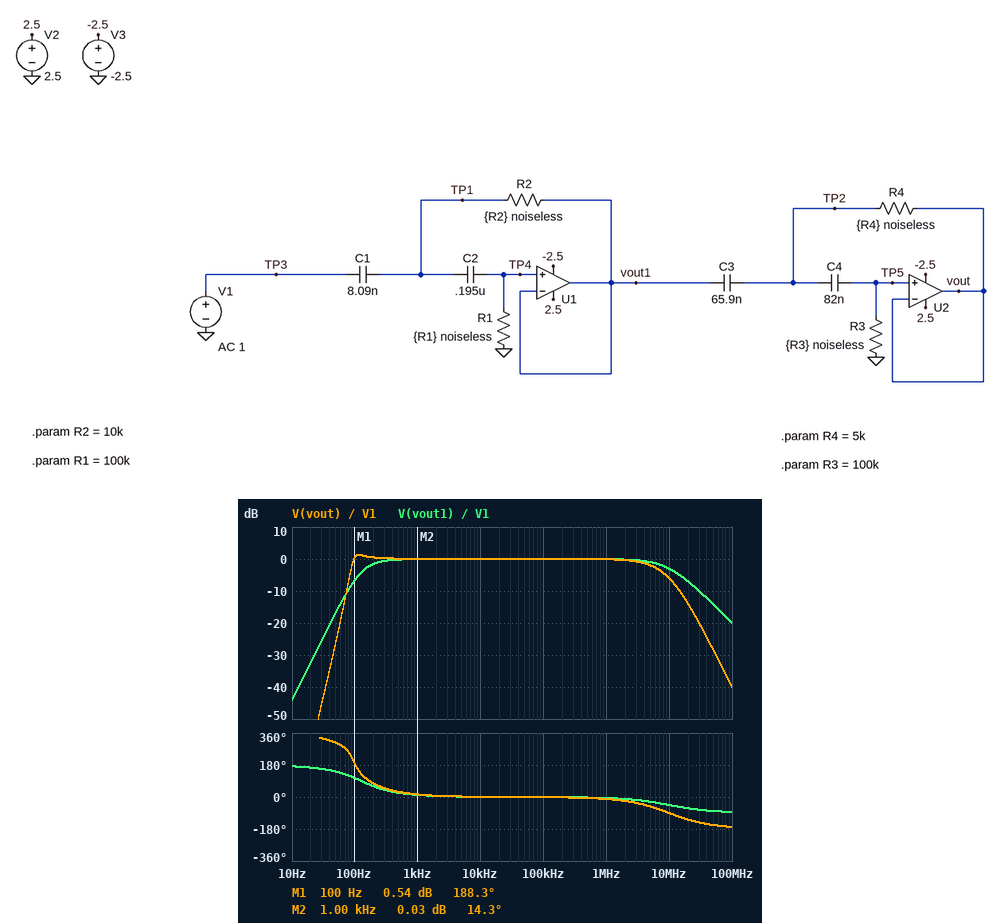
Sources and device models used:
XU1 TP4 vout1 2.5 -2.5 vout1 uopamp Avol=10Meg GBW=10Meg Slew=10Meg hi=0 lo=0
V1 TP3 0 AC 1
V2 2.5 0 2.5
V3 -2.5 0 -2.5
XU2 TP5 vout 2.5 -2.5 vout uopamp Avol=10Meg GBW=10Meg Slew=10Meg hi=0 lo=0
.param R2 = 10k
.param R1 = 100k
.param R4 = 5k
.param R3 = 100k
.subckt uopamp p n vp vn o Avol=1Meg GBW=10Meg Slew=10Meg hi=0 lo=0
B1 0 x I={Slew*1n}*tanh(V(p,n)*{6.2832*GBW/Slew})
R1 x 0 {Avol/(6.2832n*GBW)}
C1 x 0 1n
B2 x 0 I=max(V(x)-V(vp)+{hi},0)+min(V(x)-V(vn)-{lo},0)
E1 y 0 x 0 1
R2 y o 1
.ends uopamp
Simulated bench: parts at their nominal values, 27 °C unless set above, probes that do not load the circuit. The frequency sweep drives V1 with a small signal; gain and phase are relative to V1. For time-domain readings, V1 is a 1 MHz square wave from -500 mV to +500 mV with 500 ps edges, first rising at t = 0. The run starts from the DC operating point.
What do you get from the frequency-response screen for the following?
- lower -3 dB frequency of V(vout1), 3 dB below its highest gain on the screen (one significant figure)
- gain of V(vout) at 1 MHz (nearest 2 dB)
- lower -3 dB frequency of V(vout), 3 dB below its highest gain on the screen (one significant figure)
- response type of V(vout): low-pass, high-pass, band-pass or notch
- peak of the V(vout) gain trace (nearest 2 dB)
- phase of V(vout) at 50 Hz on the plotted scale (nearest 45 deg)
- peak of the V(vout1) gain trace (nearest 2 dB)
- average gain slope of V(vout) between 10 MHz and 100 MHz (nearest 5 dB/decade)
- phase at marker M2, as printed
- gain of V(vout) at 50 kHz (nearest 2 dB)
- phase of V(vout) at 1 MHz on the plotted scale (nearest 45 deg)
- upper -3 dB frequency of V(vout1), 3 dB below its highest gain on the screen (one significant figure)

100 Hz
0 dB
90 Hz
band-pass
2 dB
315 deg
0 dB
-35 dB/decade
14.3 deg
0 dB
0 deg
10 MHz
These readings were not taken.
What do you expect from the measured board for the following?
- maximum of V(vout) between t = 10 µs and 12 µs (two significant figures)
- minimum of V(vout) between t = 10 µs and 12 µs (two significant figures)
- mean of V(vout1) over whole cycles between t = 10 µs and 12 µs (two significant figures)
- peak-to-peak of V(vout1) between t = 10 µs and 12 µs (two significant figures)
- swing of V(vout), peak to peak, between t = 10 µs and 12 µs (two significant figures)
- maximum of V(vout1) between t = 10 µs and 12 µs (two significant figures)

990 mV
-9.3 mV
490 mV
1.0 V
1.0 V
990 mV
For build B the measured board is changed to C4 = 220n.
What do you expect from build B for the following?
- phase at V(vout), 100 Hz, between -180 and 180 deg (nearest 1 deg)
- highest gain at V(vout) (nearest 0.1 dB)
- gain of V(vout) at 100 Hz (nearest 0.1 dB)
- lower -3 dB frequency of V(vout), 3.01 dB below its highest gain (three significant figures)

132 deg
0 dB
-3.8 dB
114 Hz
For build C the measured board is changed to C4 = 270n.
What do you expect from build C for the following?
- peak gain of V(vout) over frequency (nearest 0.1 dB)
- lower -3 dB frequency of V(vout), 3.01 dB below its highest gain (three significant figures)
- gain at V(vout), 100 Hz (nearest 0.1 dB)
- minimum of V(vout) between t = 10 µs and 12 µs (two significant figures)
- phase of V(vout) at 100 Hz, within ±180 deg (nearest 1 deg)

0 dB
123 Hz
-4.4 dB
-8.8 mV
129 deg
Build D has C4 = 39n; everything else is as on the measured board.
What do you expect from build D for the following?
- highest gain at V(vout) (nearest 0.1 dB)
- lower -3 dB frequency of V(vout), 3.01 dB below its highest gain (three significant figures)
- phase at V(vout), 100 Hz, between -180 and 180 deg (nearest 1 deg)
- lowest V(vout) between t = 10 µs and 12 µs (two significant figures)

4.1 dB
128 Hz
-107 deg
-10 mV
